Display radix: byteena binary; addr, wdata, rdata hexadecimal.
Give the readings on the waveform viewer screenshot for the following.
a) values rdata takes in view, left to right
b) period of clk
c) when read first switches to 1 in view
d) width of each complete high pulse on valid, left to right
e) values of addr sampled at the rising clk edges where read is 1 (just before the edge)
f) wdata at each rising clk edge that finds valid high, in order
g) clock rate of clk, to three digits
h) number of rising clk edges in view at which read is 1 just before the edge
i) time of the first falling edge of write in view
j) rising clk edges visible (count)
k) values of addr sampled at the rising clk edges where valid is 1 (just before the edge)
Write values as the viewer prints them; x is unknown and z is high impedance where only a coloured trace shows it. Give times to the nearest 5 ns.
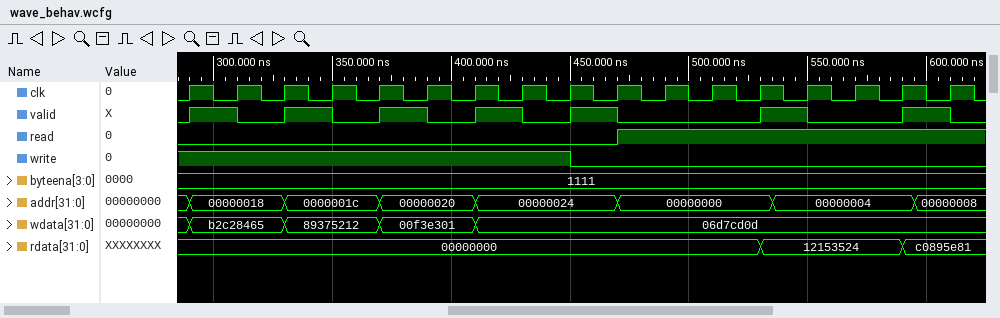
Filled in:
00000000, 12153524, c0895e81
20 ns
470 ns
20 ns, 20 ns, 20 ns, 20 ns, 20 ns, 20 ns, 20 ns
00000000, 00000000, 00000000, 00000004, 00000004, 00000004, 00000008
b2c28465, 89375212, 00f3e301, 06d7cd0d, 06d7cd0d, 06d7cd0d, 06d7cd0d
50.0 MHz
7
450 ns
17
00000018, 0000001c, 00000020, 00000024, 00000024, 00000004, 00000008
